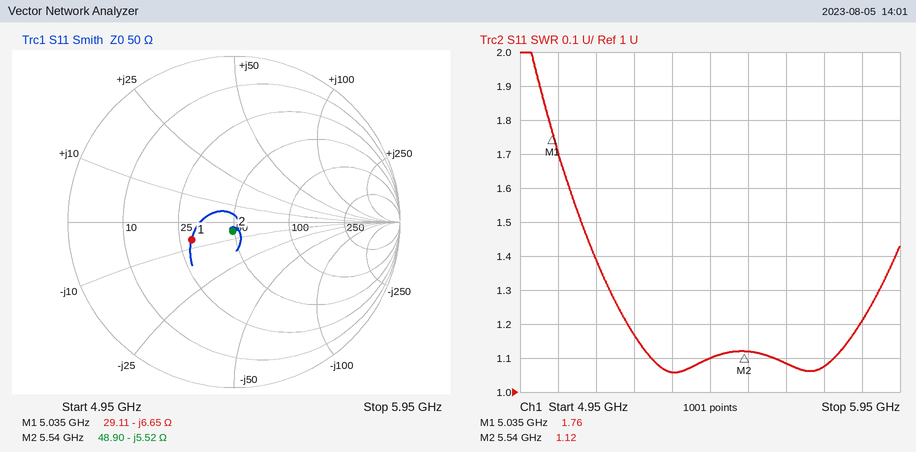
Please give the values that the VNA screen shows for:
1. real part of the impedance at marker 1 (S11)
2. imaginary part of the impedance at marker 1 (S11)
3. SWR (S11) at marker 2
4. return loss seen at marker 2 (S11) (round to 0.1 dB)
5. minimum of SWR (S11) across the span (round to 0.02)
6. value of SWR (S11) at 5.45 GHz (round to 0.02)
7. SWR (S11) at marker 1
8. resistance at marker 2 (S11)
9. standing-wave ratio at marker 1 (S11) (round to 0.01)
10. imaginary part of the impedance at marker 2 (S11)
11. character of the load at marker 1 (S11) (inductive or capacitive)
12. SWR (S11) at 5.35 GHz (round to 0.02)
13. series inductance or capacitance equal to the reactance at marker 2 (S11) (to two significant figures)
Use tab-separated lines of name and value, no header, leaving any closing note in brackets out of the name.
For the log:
real part of the impedance at marker 1	29.11 Ω
imaginary part of the impedance at marker 1	-6.65 Ω
SWR (S11) at marker 2	1.12
return loss seen at marker 2 (S11)	24.9 dB
minimum of SWR (S11) across the span	1.06
value of SWR (S11) at 5.45 GHz	1.10
SWR (S11) at marker 1	1.76
resistance at marker 2	48.90 Ω
standing-wave ratio at marker 1 (S11)	1.76
imaginary part of the impedance at marker 2	-5.52 Ω
character of the load at marker 1 (S11)	capacitive
SWR (S11) at 5.35 GHz	1.06
series inductance or capacitance equal to the reactance at marker 2 (S11)	5.2 pF
